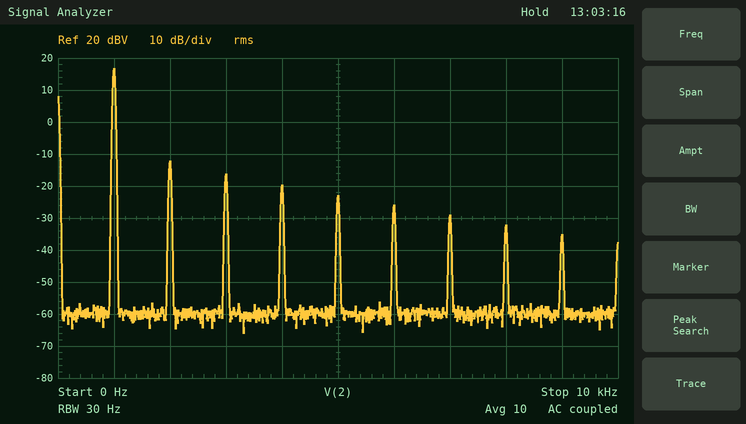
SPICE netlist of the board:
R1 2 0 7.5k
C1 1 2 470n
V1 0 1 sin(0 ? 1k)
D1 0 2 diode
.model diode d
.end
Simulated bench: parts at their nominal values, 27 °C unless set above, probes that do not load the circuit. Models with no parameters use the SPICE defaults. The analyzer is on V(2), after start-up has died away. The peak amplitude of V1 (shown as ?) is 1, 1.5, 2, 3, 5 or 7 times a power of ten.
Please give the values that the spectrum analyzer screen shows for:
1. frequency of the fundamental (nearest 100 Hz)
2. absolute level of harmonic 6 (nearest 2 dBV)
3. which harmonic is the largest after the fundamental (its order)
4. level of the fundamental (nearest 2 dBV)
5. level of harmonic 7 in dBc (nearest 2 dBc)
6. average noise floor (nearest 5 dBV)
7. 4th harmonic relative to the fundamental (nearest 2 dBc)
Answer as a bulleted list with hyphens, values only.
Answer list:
- 1.0 kHz
- -26 dBV
- 2
- 16 dBV
- -46 dBc
- -60 dBV
- -36 dBc
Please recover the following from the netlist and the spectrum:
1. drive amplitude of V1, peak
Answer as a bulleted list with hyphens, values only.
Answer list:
- 10 V
